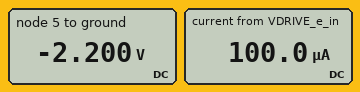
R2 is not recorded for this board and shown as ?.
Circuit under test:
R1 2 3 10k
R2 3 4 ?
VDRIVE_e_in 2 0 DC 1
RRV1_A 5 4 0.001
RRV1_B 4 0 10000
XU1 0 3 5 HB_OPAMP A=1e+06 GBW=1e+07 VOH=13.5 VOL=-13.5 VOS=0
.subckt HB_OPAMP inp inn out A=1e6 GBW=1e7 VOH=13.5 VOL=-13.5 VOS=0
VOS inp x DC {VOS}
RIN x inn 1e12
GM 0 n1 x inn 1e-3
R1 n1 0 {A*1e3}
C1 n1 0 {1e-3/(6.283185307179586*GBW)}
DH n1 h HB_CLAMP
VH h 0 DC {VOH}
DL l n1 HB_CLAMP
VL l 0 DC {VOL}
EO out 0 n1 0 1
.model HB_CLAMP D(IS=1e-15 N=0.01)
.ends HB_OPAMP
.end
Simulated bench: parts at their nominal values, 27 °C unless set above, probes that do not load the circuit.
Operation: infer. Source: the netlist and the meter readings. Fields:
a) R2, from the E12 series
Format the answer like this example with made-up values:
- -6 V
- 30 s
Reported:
- 22 kΩ
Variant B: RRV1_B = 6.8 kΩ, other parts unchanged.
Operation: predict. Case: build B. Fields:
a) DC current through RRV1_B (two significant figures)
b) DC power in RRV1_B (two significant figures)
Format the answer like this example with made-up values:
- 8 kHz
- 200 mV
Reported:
- 320 µA
- 710 µW
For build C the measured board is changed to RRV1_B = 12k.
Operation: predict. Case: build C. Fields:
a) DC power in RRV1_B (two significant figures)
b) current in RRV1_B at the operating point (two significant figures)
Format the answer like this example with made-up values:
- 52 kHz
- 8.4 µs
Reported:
- 400 µW
- 180 µA
